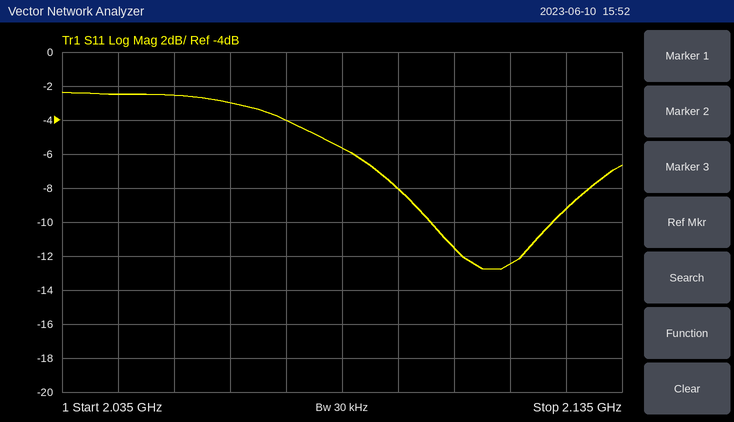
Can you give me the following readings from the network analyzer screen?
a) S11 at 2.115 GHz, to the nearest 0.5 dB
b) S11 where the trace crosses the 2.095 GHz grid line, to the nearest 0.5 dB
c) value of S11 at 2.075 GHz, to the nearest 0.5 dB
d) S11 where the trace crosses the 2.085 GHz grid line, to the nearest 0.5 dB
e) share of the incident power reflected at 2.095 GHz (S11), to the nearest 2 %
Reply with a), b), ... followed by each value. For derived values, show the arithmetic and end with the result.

a) -12.5 dB
b) -8.0 dB
c) -4.0 dB
d) -5.5 dB
e) 10^(-8/10) ≈ 16 %
